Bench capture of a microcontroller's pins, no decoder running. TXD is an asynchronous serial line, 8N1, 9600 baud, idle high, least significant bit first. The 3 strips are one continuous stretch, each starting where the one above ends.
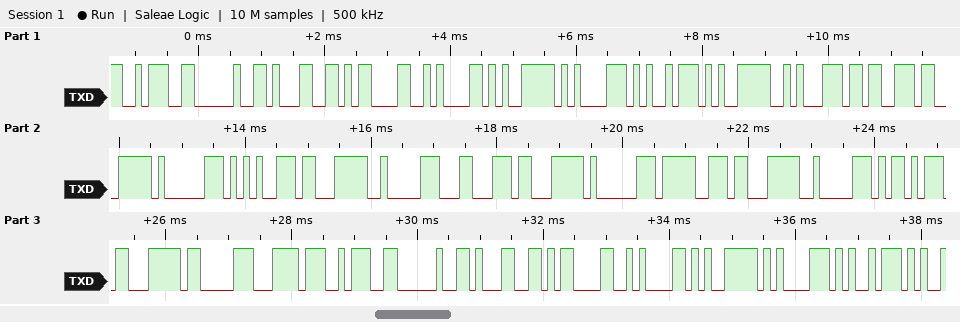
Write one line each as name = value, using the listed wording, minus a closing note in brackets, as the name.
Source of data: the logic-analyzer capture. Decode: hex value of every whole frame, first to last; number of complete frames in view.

hex value of every whole frame, first to last = 3A 20 31 0D 0A E5 85 A5 E5 8A 9B E3 81 95 E3 82 8C E3 81 9F E3 82 AD E3 83 BC 3A 20 31 0D 0A E5 85 A5
number of complete frames in view = 34
